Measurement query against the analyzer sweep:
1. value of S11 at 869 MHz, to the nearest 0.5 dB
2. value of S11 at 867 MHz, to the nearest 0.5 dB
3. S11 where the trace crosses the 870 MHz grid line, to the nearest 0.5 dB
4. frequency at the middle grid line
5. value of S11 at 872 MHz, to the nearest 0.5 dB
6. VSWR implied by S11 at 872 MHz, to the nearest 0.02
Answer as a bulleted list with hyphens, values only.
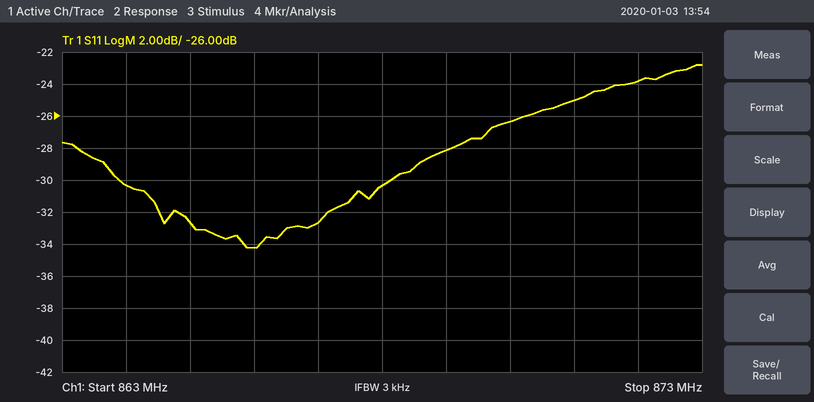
- -28.0 dB
- -32.5 dB
- -26.5 dB
- 868 MHz
- -24.0 dB
- 1.14
